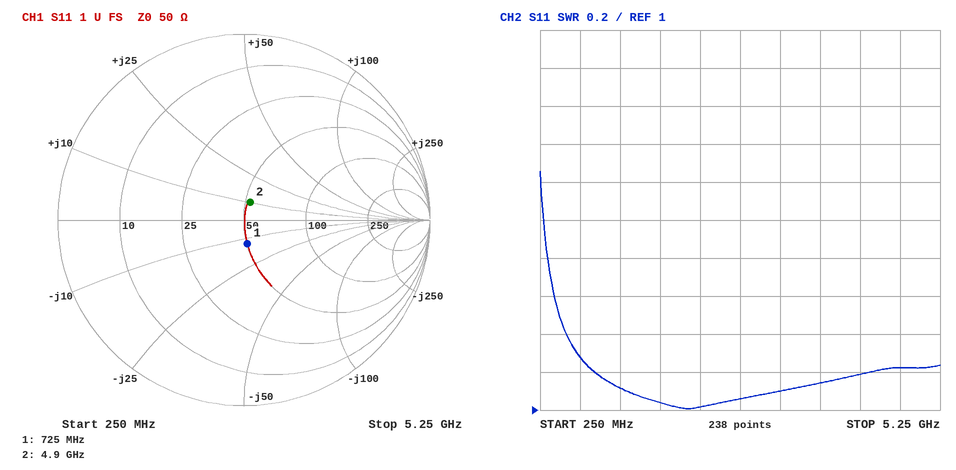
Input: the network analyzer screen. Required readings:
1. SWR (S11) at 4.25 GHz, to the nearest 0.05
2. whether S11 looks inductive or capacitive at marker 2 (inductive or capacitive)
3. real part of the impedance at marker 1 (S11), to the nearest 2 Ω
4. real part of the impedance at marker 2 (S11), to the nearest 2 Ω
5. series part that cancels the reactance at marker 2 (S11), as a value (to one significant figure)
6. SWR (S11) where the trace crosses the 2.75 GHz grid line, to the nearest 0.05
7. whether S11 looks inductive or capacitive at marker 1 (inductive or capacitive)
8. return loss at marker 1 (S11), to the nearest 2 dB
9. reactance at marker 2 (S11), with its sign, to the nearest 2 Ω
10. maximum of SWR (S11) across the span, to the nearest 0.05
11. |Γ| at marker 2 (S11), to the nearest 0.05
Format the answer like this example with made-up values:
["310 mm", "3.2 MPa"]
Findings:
["1.20", "inductive", "50 Ω", "52 Ω", "3 pF", "1.05", "capacitive", "18 dB", "+10 Ω", "2.25", "0.10"]
